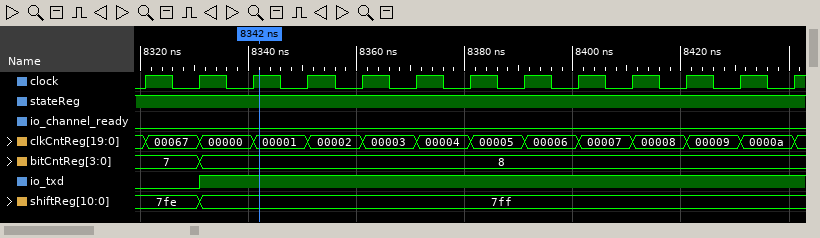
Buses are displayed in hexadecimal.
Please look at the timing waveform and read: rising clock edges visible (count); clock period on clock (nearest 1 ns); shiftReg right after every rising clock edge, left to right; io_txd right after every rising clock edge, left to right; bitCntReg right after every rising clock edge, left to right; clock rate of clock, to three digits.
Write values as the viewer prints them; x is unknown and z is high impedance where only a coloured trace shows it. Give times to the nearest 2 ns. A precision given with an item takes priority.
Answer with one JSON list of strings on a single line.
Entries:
["13", "10 ns", "7fe, 7ff, 7ff, 7ff, 7ff, 7ff, 7ff, 7ff, 7ff, 7ff, 7ff, 7ff, 7ff", "0 1 1 1 1 1 1 1 1 1 1 1 1", "7, 8, 8, 8, 8, 8, 8, 8, 8, 8, 8, 8, 8", "100 MHz"]
